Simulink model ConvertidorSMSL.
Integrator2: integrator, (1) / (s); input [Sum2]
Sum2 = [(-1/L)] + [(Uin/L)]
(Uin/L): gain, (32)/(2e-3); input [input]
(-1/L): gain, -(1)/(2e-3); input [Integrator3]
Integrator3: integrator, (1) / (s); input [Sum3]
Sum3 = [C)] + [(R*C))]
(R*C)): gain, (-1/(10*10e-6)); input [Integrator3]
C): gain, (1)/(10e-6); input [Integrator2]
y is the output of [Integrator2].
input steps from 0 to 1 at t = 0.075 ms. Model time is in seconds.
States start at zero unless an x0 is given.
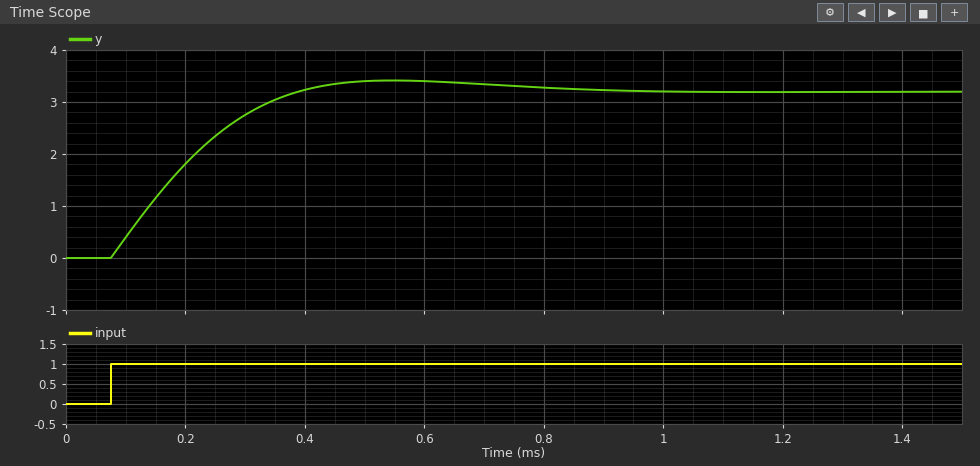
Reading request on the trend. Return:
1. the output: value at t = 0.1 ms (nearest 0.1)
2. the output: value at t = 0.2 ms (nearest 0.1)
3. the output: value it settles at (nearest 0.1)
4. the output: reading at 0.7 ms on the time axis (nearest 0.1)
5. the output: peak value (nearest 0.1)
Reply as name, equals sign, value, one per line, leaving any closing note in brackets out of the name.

the output: value at t = 0.1 ms = 0.4
the output: value at t = 0.2 ms = 1.8
the output: value it settles at = 3.2
the output: reading at 0.7 ms on the time axis = 3.3
the output: peak value = 3.4
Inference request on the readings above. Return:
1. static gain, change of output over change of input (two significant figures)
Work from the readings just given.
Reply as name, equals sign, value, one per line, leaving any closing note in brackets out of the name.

static gain, change of output over change of input = 3.2
